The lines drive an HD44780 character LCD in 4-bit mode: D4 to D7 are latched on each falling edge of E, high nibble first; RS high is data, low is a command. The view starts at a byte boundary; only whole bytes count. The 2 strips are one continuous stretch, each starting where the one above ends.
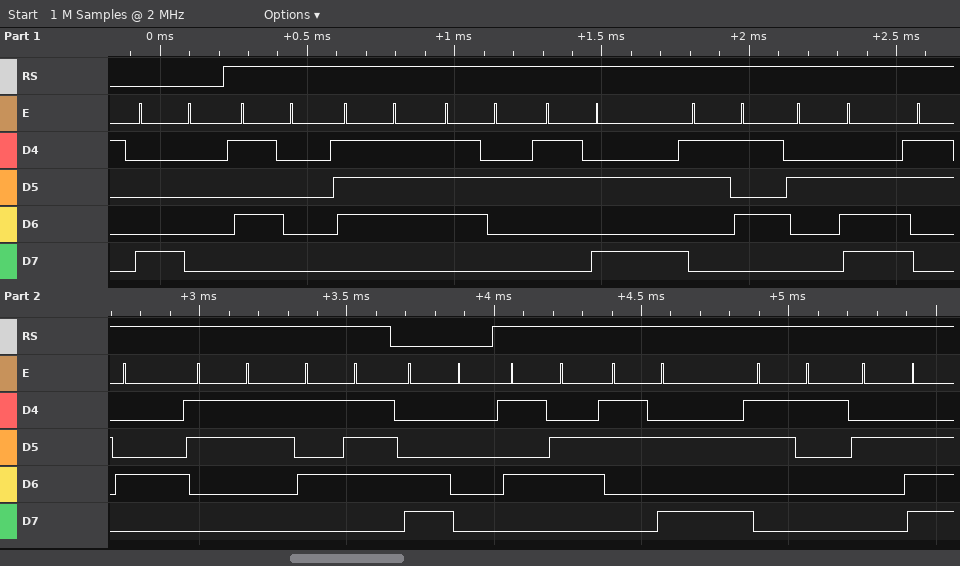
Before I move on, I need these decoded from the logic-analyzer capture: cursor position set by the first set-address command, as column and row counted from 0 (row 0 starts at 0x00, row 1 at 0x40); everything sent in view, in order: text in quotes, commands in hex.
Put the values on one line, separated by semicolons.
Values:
column 0, row 0; 0x80 "Pwr:5.43W" 0xC0 "V:1."
